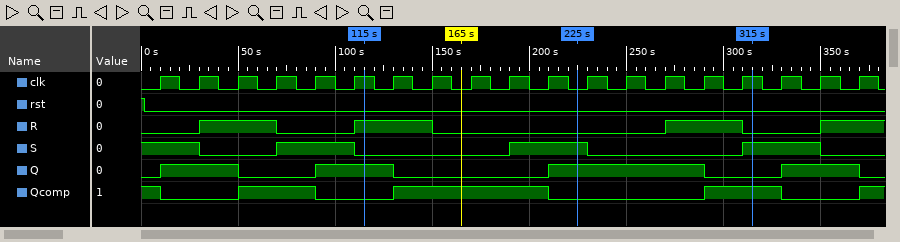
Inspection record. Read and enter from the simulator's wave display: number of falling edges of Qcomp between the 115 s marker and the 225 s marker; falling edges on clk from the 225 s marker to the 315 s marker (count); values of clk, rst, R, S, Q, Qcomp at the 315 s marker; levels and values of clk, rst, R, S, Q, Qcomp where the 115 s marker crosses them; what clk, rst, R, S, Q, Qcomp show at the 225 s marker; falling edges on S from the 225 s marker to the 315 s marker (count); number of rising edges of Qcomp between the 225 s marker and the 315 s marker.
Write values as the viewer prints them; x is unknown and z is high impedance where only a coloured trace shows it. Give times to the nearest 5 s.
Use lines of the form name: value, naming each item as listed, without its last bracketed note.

number of falling edges of Qcomp between the 115 s marker and the 225 s marker: 1
falling edges on clk from the 225 s marker to the 315 s marker: 4
values of clk, rst, R, S, Q, Qcomp at the 315 s marker: clk=1, rst=0, R=0, S=1, Q=0, Qcomp=1
levels and values of clk, rst, R, S, Q, Qcomp where the 115 s marker crosses them: clk=1, rst=0, R=1, S=0, Q=1, Qcomp=0
what clk, rst, R, S, Q, Qcomp show at the 225 s marker: clk=0, rst=0, R=0, S=1, Q=1, Qcomp=0
falling edges on S from the 225 s marker to the 315 s marker: 1
number of rising edges of Qcomp between the 225 s marker and the 315 s marker: 1
